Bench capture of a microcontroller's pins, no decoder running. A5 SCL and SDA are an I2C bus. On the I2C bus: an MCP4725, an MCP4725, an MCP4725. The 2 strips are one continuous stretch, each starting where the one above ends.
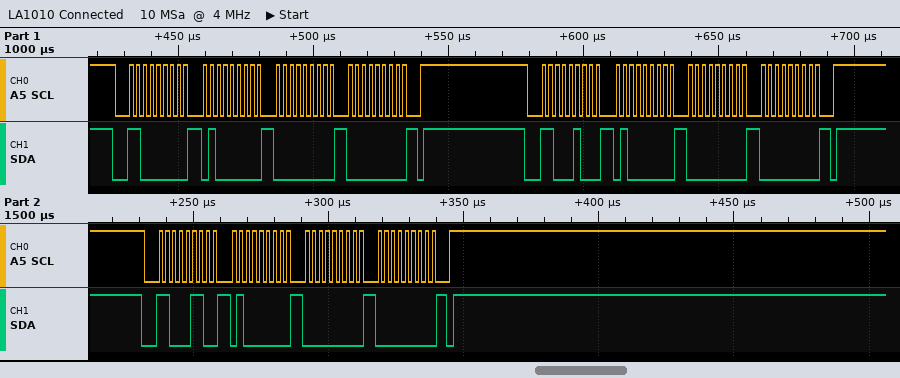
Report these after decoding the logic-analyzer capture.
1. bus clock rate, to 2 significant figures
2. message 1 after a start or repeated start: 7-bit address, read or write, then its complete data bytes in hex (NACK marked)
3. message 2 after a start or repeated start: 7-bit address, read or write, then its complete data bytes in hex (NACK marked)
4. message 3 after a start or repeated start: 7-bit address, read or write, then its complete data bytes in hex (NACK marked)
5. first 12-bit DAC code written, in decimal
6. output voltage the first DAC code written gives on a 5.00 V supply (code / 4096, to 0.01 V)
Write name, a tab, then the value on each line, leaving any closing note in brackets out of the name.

bus clock rate, to 2 significant figures	400 kHz
message 1 after a start or repeated start: 7-bit address, read or write, then its complete data bytes in hex	0x60 write: 40 00 00
message 2 after a start or repeated start: 7-bit address, read or write, then its complete data bytes in hex	0x62 write: 40 00 00
message 3 after a start or repeated start: 7-bit address, read or write, then its complete data bytes in hex	0x63 write: 40 00 00
first 12-bit DAC code written, in decimal	0
output voltage the first DAC code written gives on a 5.00 V supply	0.00 V
